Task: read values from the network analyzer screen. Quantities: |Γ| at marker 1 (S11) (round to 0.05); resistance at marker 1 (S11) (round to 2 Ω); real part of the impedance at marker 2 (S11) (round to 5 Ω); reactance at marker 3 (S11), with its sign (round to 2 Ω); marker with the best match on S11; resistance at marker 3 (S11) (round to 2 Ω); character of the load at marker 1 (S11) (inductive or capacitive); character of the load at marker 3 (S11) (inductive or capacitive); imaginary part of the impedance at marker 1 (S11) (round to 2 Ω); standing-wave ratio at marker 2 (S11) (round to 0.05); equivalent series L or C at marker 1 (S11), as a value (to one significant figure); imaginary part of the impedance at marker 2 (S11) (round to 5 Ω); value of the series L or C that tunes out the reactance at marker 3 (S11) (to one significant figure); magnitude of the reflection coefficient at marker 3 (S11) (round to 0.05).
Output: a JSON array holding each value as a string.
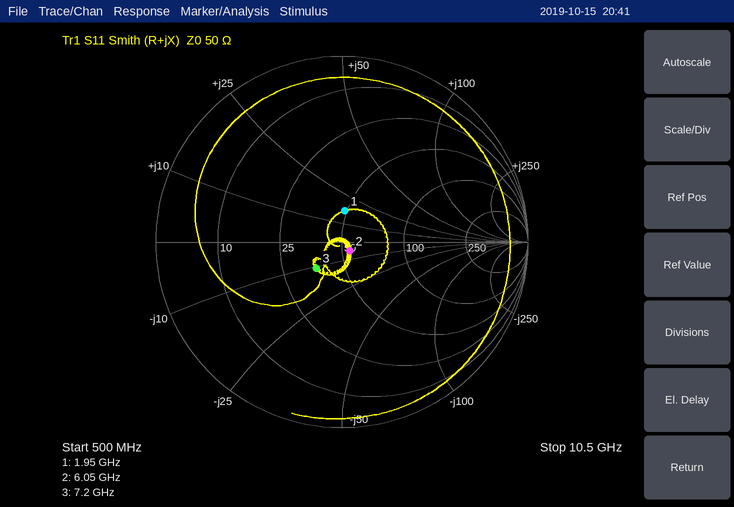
["0.15", "48 Ω", "55 Ω", "-10 Ω", "marker 2", "36 Ω", "inductive", "capacitive", "+16 Ω", "1.15", "1 nH", "-5 Ω", "200 pH", "0.20"]
